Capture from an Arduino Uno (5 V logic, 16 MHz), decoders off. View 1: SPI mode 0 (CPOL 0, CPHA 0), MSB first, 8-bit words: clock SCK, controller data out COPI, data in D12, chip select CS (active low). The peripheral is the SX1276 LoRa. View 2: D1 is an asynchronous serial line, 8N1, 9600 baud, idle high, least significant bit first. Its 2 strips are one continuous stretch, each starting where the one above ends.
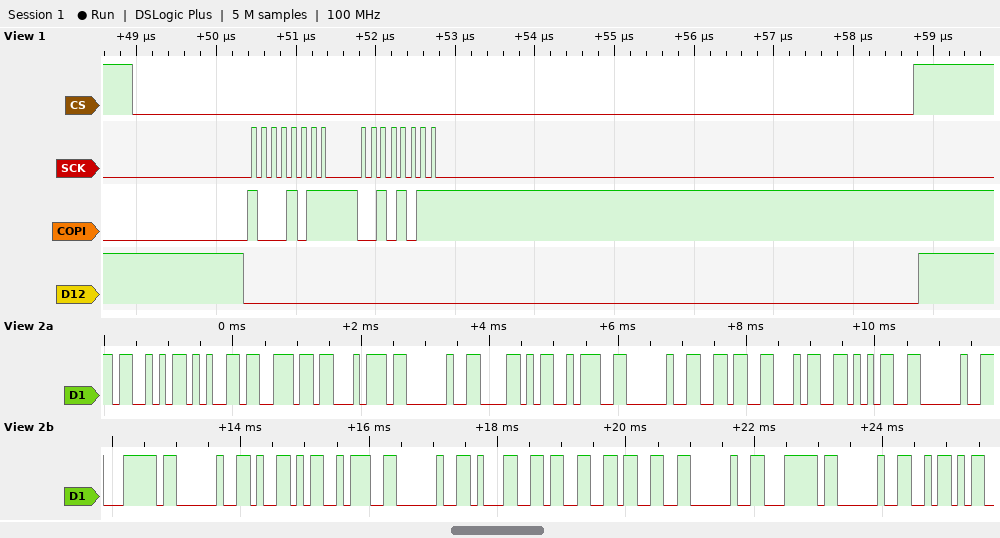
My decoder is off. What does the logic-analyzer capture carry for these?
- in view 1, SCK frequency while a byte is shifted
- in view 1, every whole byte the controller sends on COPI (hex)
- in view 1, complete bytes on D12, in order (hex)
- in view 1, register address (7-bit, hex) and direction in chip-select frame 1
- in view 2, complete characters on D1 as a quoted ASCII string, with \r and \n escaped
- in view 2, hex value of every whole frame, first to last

8 MHz
8B 2B
00 00
0x0B write
"Sent X: 645 | Y: 133 | Z"
53 65 6E 74 20 58 3A 20 36 34 35 20 7C 20 59 3A 20 31 33 33 20 7C 20 5A
